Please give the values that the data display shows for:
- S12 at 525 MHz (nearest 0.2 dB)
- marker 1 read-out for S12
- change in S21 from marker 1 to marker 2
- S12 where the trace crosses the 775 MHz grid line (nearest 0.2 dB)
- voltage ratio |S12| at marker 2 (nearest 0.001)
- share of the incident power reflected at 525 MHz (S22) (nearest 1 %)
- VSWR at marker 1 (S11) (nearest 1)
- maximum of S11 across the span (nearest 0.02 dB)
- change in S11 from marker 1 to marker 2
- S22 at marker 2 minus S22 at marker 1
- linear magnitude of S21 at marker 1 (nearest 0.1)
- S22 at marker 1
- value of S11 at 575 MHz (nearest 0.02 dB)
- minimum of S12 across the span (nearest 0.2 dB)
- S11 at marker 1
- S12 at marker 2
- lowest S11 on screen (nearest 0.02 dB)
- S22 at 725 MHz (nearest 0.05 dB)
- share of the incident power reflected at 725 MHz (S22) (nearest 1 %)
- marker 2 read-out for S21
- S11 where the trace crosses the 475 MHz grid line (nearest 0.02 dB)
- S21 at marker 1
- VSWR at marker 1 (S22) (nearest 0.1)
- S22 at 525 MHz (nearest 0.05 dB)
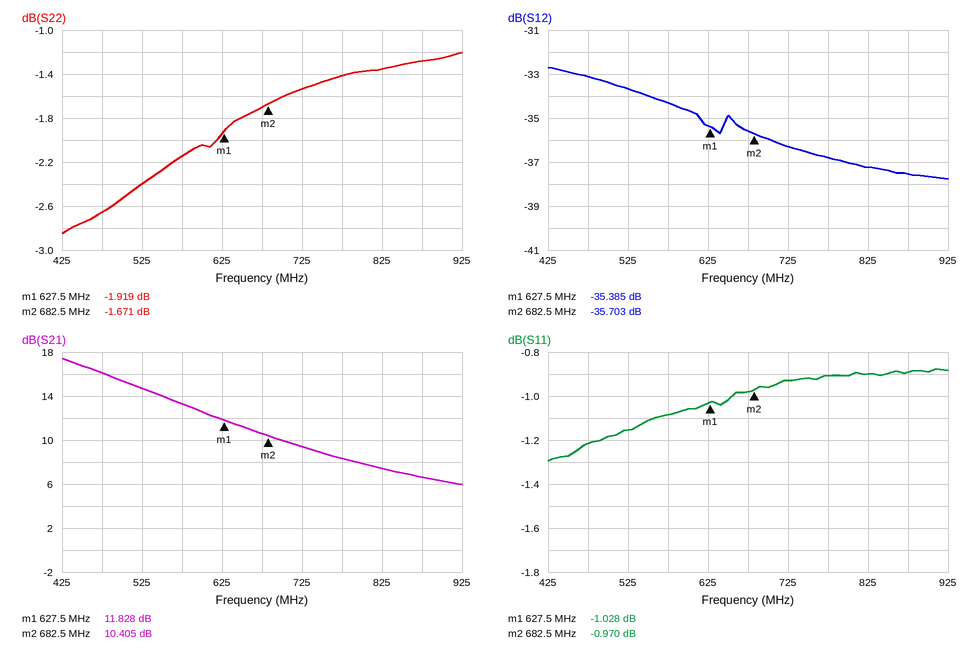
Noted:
-33.6 dB
-35.385 dB
-1.423 dB
-36.8 dB
0.016
58 %
17
-0.88 dB
0.058 dB
0.248 dB
3.9
-1.919 dB
-1.08 dB
-37.8 dB
-1.028 dB
-35.703 dB
-1.30 dB
-1.55 dB
70 %
10.405 dB
-1.22 dB
11.828 dB
9.1
-2.40 dB
